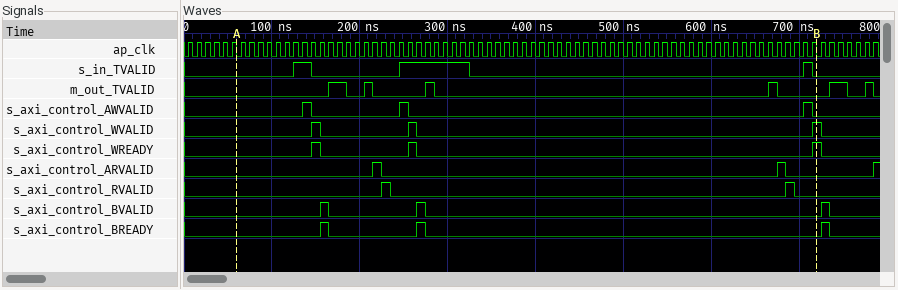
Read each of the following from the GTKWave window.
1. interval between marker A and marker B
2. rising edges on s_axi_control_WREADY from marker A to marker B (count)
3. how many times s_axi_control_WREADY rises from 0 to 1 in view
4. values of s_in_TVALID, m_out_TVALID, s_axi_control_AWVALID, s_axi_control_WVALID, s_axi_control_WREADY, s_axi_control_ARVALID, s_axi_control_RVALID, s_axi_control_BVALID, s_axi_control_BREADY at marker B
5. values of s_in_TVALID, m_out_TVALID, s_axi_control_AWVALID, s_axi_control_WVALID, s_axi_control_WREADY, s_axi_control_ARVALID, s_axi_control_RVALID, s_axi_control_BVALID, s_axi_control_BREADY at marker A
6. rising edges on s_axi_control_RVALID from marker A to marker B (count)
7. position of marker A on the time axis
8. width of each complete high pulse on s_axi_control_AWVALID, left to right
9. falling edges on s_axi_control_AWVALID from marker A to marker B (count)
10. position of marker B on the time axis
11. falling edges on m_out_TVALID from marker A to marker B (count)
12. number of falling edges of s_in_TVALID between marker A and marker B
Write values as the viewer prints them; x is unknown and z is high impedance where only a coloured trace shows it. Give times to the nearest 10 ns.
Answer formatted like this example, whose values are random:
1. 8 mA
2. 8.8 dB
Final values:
1. 660 ns
2. 3
3. 3
4. s_in_TVALID=0, m_out_TVALID=0, s_axi_control_AWVALID=0, s_axi_control_WVALID=1, s_axi_control_WREADY=1, s_axi_control_ARVALID=0, s_axi_control_RVALID=0, s_axi_control_BVALID=0, s_axi_control_BREADY=0
5. s_in_TVALID=0, m_out_TVALID=0, s_axi_control_AWVALID=0, s_axi_control_WVALID=0, s_axi_control_WREADY=0, s_axi_control_ARVALID=0, s_axi_control_RVALID=0, s_axi_control_BVALID=0, s_axi_control_BREADY=0
6. 2
7. 60 ns
8. 10 ns, 10 ns, 10 ns
9. 3
10. 720 ns
11. 4
12. 3
